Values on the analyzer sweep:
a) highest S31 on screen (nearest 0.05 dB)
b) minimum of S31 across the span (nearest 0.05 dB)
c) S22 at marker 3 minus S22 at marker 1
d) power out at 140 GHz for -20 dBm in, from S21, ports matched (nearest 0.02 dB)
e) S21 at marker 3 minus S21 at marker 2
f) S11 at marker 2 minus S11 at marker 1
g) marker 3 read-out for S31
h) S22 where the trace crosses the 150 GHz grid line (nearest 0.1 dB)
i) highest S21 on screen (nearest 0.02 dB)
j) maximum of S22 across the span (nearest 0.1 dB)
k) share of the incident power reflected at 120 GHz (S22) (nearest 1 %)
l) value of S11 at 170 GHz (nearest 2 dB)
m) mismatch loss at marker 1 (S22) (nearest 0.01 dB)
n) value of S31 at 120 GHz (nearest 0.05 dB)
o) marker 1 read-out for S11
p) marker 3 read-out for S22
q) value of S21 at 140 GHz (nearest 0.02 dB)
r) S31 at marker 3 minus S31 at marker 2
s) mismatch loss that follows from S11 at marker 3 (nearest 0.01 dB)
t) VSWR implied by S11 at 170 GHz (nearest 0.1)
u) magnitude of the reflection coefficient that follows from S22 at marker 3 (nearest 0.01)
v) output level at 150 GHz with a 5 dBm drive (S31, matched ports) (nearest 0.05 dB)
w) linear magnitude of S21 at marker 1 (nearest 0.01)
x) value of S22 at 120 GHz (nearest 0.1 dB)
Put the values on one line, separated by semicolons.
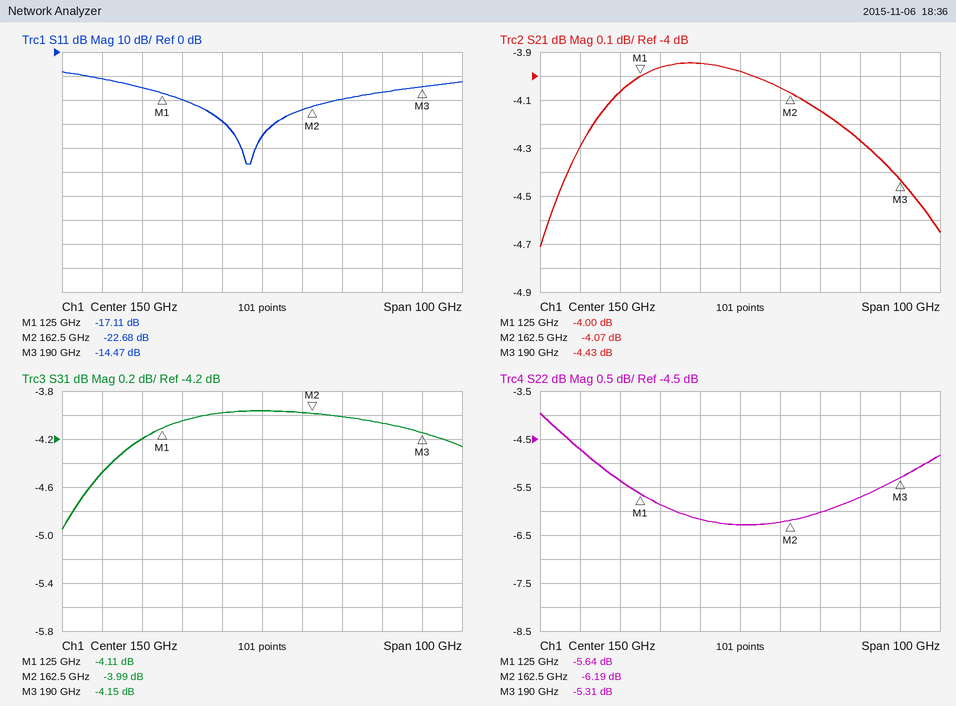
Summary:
-3.95 dB; -4.95 dB; 0.33 dB; -23.94 dBm; -0.36 dB; -5.57 dB; -4.15 dB; -6.3 dB; -3.94 dB; -4.0 dB; 29 %; -20 dB; 1.38 dB; -4.20 dB; -17.11 dB; -5.31 dB; -3.94 dB; -0.16 dB; 0.16 dB; 1.2; 0.54; 1.05 dBm; 0.63; -5.4 dB
